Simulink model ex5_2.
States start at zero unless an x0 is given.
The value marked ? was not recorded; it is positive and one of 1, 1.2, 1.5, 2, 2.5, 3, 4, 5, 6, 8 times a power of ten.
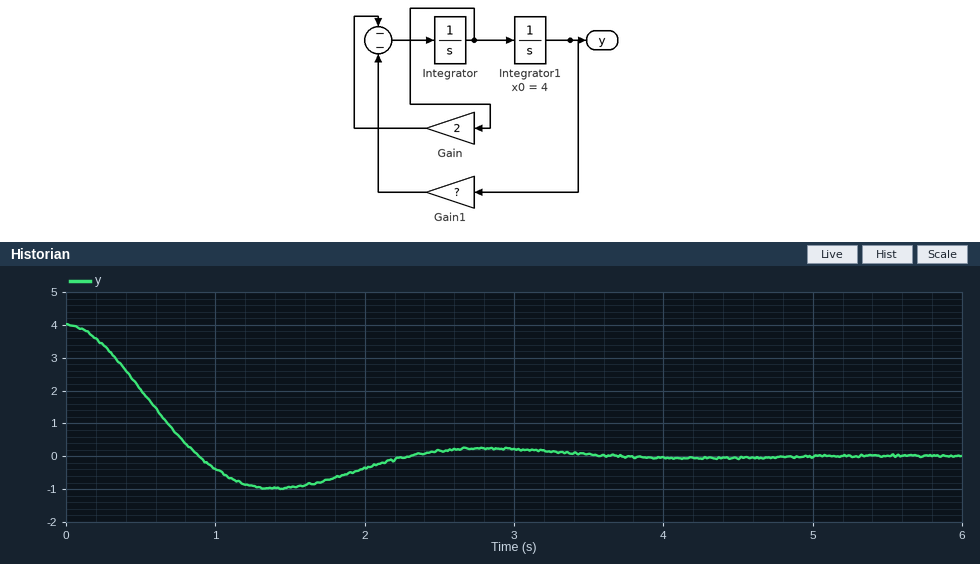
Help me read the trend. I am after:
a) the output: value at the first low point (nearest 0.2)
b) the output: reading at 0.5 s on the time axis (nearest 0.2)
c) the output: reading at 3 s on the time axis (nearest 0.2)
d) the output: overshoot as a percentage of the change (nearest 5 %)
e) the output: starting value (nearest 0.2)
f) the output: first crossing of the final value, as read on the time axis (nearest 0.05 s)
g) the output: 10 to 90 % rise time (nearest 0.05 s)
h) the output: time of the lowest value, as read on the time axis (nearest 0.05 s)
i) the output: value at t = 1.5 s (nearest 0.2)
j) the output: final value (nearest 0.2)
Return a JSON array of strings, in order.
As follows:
["-1.0", "2.0", "0.2", "25 %", "4.0", "0.90 s", "0.60 s", "1.40 s", "-1.0", "0.0"]
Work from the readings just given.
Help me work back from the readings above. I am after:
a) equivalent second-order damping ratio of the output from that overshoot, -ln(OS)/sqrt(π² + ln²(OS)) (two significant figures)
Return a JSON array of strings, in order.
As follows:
["0.40"]
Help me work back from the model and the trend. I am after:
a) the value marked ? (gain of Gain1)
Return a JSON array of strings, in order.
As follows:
["6"]
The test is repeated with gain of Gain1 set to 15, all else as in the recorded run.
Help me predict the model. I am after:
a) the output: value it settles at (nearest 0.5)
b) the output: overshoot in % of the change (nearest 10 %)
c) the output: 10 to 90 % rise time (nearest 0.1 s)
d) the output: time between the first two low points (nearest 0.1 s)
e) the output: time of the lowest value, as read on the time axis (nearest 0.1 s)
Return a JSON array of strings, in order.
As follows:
["0.0", "40 %", "0.3 s", "1.7 s", "0.8 s"]
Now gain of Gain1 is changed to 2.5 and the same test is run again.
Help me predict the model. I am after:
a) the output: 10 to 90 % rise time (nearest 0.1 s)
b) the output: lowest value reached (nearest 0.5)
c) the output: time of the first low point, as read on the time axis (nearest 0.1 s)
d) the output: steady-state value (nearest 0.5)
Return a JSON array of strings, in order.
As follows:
["1.2 s", "-0.5", "2.6 s", "0.0"]
